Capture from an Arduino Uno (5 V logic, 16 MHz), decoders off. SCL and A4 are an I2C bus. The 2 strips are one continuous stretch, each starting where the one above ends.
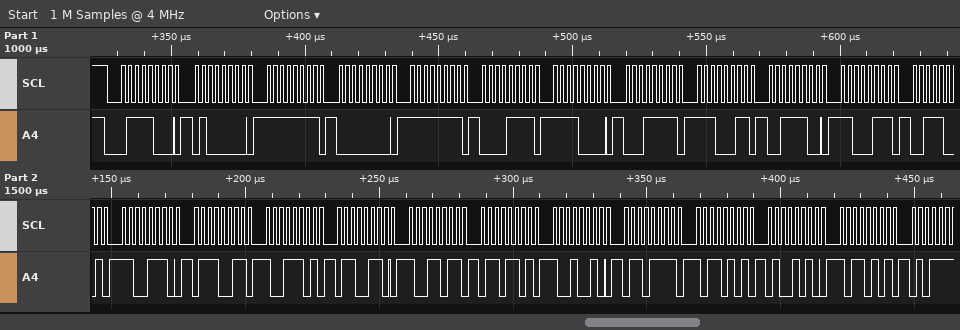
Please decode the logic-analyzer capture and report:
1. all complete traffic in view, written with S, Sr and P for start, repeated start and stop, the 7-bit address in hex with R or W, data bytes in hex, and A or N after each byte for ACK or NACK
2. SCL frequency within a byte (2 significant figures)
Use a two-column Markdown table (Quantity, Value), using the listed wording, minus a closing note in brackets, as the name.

| Quantity | Value |
|---|---|
| all complete traffic in view, written with S, Sr and P for start, repeated start and stop, the 7-bit address in hex with R or W, data bytes in hex, and A or N after each byte for ACK or NACK | S 3CW A 40 A FF A 00 A FF A 0F A F0 A 1F A E3 A 3C A C7 A 39 A CE A 73 A 9D A 66 A 9B A 6D A 92 A 6F A B5 A 4A A B5 A |
| SCL frequency within a byte | 400 kHz |
